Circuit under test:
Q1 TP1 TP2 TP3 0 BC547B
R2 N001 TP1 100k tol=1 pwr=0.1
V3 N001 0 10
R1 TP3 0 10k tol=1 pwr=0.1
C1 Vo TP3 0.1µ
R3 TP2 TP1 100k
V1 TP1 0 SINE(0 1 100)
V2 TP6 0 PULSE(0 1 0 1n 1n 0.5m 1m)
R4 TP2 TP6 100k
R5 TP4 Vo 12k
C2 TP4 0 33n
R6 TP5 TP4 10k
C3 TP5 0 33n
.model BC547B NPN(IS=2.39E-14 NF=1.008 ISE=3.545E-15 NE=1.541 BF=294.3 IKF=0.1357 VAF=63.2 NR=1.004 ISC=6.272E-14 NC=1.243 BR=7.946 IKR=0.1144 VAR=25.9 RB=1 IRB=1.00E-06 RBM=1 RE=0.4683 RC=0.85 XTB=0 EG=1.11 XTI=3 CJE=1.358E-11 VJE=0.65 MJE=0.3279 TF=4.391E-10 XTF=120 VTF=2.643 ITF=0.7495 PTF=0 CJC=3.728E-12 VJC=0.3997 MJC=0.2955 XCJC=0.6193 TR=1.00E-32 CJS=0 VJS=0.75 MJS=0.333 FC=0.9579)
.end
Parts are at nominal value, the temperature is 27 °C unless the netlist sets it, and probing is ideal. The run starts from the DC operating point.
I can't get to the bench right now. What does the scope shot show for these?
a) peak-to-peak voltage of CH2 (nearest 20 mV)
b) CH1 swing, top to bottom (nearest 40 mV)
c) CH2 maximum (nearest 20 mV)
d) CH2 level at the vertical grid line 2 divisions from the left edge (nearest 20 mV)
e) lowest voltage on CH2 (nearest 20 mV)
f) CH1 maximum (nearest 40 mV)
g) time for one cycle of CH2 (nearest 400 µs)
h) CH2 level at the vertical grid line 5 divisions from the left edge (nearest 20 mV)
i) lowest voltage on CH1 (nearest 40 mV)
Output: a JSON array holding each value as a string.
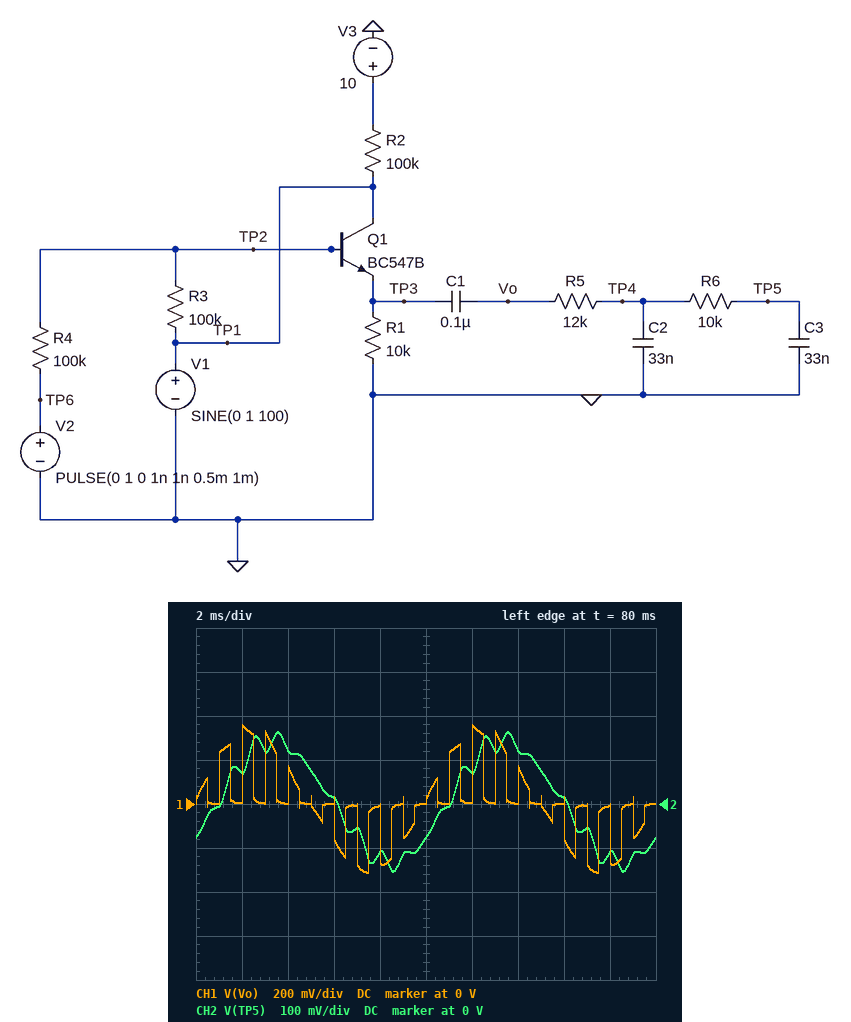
["320 mV", "680 mV", "160 mV", "120 mV", "-160 mV", "360 mV", "10.0 ms", "-80 mV", "-320 mV"]
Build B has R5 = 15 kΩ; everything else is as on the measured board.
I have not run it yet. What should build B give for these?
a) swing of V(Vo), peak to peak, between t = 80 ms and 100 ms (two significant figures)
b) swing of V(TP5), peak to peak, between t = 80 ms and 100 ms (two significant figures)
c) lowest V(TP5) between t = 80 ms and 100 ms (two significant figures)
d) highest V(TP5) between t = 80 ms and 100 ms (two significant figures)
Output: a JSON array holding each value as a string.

["690 mV", "300 mV", "-150 mV", "150 mV"]
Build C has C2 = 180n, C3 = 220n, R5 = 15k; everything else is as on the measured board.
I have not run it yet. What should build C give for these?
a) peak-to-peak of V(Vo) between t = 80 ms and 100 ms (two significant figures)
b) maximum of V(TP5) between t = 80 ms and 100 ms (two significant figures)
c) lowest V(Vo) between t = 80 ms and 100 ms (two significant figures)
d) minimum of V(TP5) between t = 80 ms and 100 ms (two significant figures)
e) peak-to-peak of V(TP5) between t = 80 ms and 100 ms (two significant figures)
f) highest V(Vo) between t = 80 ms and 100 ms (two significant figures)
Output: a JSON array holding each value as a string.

["660 mV", "30 mV", "-300 mV", "-25 mV", "55 mV", "360 mV"]
